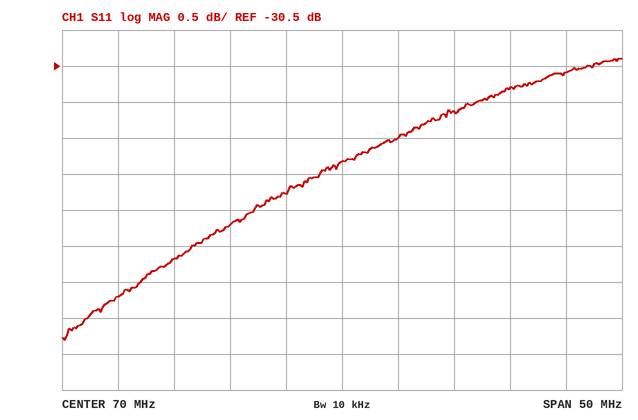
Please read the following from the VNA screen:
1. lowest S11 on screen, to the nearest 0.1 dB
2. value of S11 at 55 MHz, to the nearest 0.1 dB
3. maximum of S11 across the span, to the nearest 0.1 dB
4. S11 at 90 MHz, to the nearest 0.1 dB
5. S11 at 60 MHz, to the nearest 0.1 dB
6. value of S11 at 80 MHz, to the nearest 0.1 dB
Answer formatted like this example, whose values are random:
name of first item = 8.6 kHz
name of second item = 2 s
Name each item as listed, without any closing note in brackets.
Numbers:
lowest S11 on screen, to the nearest 0.1 dB = -34.3 dB
value of S11 at 55 MHz, to the nearest 0.1 dB = -33.2 dB
maximum of S11 across the span, to the nearest 0.1 dB = -30.4 dB
S11 at 90 MHz, to the nearest 0.1 dB = -30.6 dB
S11 at 60 MHz, to the nearest 0.1 dB = -32.7 dB
value of S11 at 80 MHz, to the nearest 0.1 dB = -31.1 dB
